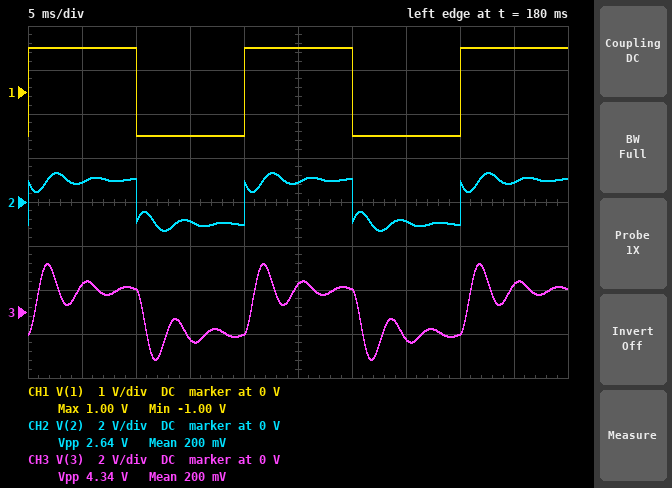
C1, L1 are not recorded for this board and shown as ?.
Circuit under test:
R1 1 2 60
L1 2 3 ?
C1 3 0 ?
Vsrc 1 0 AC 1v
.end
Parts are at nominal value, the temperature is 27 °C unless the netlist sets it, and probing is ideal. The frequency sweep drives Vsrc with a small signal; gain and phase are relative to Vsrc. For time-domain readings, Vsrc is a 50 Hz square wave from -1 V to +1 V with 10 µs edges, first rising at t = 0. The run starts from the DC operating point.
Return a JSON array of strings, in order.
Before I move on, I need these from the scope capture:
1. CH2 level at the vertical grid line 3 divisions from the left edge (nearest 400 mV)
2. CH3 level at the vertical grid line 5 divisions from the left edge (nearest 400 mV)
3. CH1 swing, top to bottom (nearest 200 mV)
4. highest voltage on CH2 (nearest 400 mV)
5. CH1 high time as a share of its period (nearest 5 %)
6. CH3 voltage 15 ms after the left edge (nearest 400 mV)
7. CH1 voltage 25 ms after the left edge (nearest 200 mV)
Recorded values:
["-800 mV", "1.2 V", "2.0 V", "1.2 V", "50 %", "-1.2 V", "1.0 V"]
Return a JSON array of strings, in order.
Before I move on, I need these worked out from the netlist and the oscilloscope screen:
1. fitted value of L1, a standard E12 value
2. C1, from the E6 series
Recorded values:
["100 mH", "3.3 µF"]
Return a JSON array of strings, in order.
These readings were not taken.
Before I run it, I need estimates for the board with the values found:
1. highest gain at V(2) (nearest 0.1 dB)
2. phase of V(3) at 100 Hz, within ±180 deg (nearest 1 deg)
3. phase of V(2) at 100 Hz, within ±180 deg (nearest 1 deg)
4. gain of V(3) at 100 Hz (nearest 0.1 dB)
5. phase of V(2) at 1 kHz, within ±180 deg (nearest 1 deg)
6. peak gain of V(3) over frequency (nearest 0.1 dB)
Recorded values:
["0 dB", "-8 deg", "-8 deg", "1.1 dB", "6 deg", "9.4 dB"]
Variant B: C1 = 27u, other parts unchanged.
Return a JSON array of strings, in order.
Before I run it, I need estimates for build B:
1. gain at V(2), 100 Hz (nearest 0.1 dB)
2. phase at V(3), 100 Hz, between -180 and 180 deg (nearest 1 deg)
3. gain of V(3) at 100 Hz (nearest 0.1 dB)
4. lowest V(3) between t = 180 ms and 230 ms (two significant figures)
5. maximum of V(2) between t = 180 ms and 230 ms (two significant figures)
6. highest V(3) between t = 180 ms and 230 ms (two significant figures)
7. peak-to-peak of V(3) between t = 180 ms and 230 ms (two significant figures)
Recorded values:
["-23.8 dB", "-94 deg", "-0.2 dB", "-1.3 V", "1.2 V", "1.3 V", "2.7 V"]
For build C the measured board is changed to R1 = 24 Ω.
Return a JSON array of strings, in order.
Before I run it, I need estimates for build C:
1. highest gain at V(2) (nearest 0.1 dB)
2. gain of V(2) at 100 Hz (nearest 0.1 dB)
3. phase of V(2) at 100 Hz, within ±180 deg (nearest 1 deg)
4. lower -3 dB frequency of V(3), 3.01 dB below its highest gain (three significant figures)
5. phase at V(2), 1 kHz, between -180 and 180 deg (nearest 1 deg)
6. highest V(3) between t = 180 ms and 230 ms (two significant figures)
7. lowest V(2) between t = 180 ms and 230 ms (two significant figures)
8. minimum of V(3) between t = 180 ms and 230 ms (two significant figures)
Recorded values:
["0 dB", "0 dB", "-3 deg", "256 Hz", "2 deg", "2.5 V", "-1.2 V", "-2.5 V"]
